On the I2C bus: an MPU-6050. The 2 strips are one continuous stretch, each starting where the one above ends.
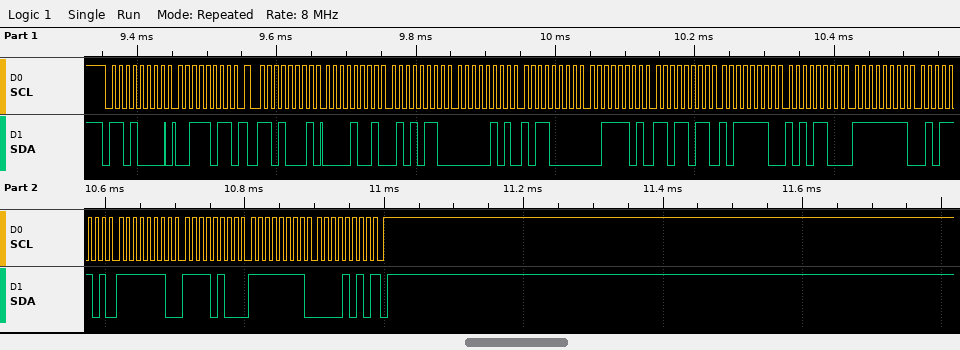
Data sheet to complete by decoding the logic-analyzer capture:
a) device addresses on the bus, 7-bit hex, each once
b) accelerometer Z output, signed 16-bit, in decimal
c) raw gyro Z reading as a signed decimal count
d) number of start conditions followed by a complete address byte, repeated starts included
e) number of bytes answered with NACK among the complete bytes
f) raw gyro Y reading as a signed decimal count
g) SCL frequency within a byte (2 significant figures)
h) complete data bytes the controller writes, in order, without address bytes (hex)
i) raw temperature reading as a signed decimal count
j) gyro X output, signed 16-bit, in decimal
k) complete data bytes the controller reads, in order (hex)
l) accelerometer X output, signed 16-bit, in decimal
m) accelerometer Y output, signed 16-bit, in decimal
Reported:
0x68
15835
-246
2
1
-268
100 kHz
3B
-16724
-163
09 56 05 B0 3D DB BE AC FF 5D FE F4 FF 0A
2390
1456
